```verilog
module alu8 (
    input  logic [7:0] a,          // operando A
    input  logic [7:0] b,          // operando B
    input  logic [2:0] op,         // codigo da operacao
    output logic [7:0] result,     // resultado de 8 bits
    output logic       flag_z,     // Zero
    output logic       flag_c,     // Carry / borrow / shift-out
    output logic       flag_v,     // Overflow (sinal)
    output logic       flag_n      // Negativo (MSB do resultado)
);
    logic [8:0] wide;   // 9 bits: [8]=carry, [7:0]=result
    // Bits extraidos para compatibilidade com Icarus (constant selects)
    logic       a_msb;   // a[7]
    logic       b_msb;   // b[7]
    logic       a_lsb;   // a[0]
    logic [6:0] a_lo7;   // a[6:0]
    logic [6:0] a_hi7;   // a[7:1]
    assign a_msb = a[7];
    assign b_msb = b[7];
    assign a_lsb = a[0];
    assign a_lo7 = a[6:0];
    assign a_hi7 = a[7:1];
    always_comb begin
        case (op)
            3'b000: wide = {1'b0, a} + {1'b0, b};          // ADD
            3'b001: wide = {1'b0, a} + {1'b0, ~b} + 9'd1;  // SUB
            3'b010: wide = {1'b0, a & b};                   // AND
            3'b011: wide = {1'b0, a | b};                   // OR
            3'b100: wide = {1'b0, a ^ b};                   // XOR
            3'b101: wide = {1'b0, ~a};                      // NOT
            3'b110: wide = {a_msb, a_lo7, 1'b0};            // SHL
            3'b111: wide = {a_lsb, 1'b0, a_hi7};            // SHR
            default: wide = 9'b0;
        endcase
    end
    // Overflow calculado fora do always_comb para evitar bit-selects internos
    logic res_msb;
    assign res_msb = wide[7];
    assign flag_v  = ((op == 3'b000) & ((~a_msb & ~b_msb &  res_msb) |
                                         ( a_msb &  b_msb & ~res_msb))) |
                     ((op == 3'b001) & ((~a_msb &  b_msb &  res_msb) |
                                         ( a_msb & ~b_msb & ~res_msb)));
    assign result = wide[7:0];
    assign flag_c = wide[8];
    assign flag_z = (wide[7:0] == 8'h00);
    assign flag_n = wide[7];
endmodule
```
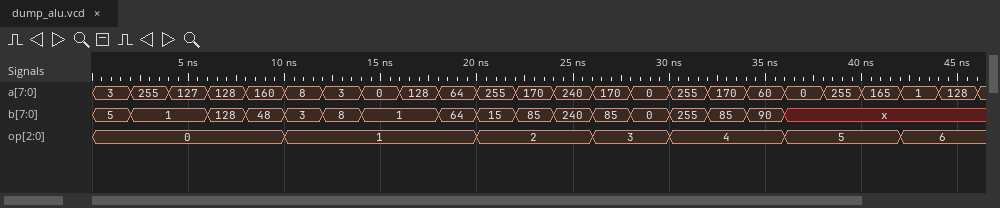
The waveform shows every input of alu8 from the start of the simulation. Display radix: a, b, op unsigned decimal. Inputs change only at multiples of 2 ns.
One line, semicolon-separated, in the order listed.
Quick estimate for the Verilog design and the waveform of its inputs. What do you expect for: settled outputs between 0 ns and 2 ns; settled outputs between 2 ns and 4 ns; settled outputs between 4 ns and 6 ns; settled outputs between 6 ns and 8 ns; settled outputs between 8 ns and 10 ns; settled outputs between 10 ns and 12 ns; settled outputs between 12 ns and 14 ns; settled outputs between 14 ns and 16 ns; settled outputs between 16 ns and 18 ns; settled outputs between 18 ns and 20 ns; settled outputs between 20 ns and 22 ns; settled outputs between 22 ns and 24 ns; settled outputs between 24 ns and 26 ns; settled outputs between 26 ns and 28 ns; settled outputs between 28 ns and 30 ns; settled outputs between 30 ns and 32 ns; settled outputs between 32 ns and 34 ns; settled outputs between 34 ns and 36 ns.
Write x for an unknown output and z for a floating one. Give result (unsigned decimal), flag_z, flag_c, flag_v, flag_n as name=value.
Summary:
result=8, flag_z=0, flag_c=0, flag_v=0, flag_n=0; result=0, flag_z=1, flag_c=1, flag_v=0, flag_n=0; result=128, flag_z=0, flag_c=0, flag_v=1, flag_n=1; result=0, flag_z=1, flag_c=1, flag_v=1, flag_n=0; result=208, flag_z=0, flag_c=0, flag_v=0, flag_n=1; result=5, flag_z=0, flag_c=1, flag_v=0, flag_n=0; result=251, flag_z=0, flag_c=0, flag_v=0, flag_n=1; result=255, flag_z=0, flag_c=0, flag_v=0, flag_n=1; result=127, flag_z=0, flag_c=1, flag_v=1, flag_n=0; result=0, flag_z=1, flag_c=1, flag_v=0, flag_n=0; result=15, flag_z=0, flag_c=0, flag_v=0, flag_n=0; result=0, flag_z=1, flag_c=0, flag_v=0, flag_n=0; result=240, flag_z=0, flag_c=0, flag_v=0, flag_n=1; result=255, flag_z=0, flag_c=0, flag_v=0, flag_n=1; result=0, flag_z=1, flag_c=0, flag_v=0, flag_n=0; result=0, flag_z=1, flag_c=0, flag_v=0, flag_n=0; result=255, flag_z=0, flag_c=0, flag_v=0, flag_n=1; result=102, flag_z=0, flag_c=0, flag_v=0, flag_n=0
